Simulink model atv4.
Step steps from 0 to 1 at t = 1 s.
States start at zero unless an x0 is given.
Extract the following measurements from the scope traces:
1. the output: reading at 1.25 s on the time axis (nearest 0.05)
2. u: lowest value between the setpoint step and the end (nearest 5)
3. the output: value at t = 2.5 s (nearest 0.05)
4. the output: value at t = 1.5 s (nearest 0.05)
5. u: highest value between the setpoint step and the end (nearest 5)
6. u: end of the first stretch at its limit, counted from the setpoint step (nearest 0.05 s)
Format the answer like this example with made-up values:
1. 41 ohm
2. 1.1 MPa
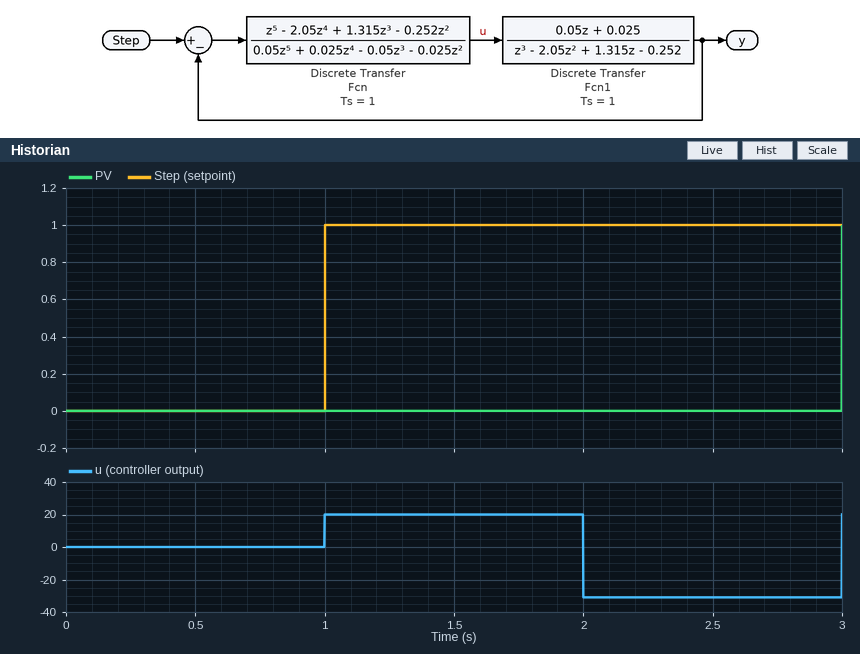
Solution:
1. 0.00
2. -30
3. 0.00
4. 0.00
5. 20
6. 1.00 s
